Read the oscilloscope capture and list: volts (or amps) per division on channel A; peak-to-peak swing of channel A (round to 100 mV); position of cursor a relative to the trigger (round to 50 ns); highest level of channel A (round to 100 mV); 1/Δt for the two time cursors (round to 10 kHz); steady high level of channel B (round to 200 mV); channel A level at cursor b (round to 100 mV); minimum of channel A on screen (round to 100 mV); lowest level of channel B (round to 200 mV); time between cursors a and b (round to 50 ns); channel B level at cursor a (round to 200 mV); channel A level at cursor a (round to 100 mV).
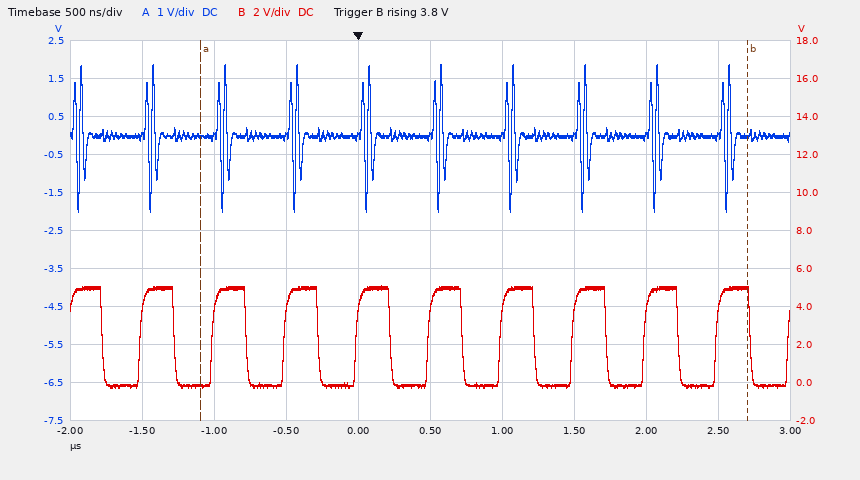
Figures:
1 V
3.9 V
-1.10 µs
1.9 V
260 kHz
5.0 V
100 mV
-2.0 V
-200 mV
3.80 µs
-200 mV
0.0 V
